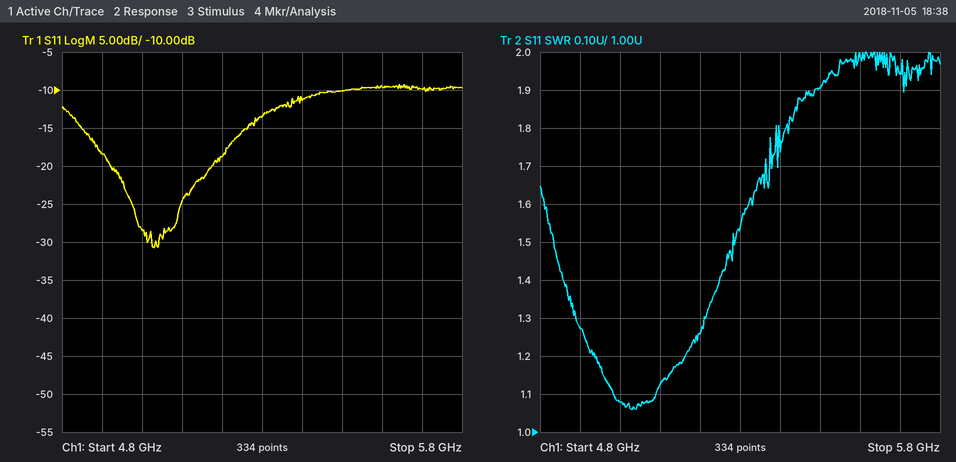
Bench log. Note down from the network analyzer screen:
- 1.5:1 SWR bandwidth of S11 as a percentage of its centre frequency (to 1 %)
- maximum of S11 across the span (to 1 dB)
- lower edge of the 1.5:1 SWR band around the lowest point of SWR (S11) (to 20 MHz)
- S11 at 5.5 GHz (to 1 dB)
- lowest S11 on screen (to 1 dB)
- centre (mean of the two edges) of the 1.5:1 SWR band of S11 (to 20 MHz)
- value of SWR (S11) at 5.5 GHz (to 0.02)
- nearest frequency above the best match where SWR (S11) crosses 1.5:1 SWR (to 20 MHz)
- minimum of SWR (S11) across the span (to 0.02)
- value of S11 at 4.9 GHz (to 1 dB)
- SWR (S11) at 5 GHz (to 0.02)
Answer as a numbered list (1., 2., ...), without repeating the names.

1. 9 %
2. -9 dB
3. 4.84 GHz
4. -10 dB
5. -31 dB
6. 5.06 GHz
7. 1.90
8. 5.28 GHz
9. 1.06
10. -18 dB
11. 1.08
